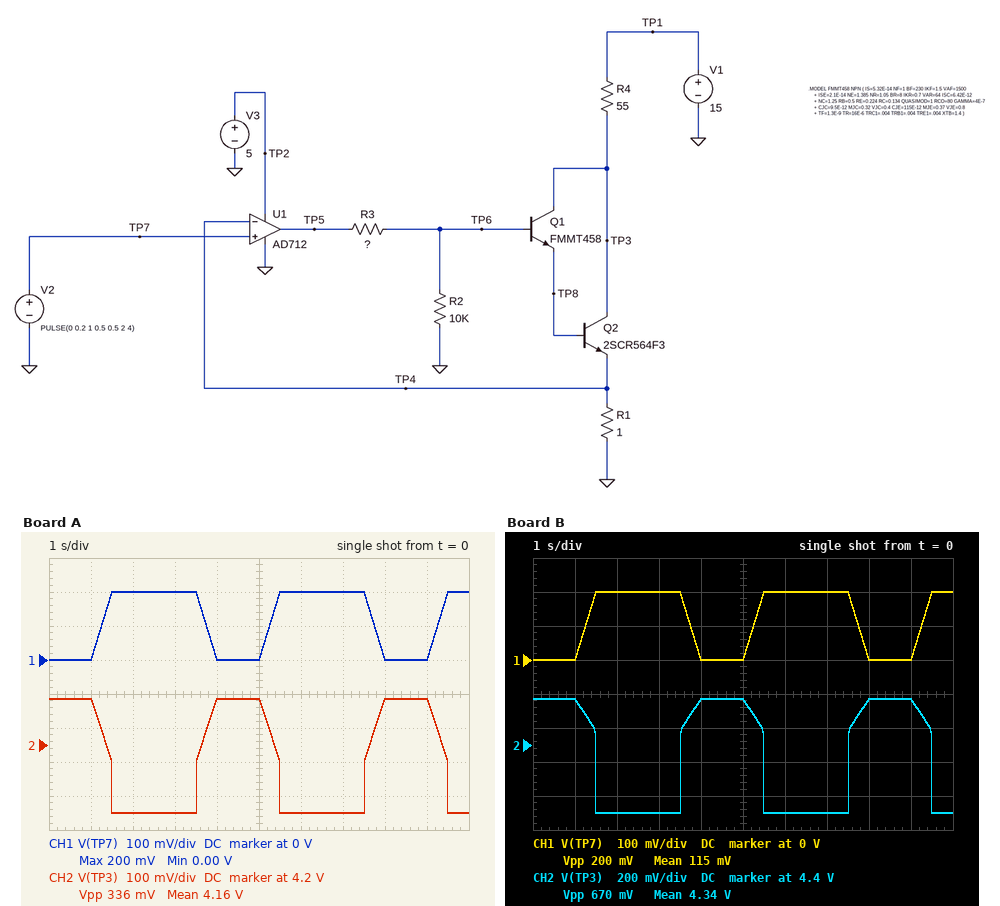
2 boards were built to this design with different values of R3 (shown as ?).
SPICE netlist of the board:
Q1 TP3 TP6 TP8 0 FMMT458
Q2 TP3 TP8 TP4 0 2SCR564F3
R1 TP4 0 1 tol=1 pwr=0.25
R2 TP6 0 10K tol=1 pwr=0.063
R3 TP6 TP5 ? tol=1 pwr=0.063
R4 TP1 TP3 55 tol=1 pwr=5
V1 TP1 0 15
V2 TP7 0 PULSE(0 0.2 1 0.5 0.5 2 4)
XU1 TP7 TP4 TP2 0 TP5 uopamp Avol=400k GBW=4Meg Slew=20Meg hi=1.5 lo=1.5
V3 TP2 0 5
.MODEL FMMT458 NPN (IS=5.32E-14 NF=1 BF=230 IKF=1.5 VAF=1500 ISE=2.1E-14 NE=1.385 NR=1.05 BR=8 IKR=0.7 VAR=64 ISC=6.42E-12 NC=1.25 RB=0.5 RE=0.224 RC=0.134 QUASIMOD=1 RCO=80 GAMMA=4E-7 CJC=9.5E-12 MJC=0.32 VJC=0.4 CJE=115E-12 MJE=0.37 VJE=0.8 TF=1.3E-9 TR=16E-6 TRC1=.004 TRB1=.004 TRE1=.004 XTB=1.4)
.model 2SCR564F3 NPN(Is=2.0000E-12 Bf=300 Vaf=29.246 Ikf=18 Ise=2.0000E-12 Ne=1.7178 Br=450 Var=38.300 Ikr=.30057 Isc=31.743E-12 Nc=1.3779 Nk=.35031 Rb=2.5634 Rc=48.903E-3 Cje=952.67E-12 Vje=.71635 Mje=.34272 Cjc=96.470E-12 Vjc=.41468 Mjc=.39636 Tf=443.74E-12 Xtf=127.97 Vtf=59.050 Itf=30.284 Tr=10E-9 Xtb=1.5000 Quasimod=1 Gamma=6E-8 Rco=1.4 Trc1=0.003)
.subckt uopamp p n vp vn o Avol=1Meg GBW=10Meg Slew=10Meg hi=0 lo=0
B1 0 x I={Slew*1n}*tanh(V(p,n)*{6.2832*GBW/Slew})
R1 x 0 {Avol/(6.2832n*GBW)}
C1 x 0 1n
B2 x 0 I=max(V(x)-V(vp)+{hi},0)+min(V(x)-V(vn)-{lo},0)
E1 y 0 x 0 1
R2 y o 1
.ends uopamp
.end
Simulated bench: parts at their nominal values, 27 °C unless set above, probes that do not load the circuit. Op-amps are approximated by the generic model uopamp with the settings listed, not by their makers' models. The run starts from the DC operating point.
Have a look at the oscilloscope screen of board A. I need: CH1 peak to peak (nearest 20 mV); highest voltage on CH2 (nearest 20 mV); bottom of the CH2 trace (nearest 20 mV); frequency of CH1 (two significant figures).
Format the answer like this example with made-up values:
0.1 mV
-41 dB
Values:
200 mV
4.34 V
4.00 V
250 mHz
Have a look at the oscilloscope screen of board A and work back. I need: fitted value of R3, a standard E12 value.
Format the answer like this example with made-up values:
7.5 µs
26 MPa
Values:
330 Ω
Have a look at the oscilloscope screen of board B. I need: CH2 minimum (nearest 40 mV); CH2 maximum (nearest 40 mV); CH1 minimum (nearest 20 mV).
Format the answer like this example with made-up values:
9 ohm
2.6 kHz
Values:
4.00 V
4.68 V
0 V
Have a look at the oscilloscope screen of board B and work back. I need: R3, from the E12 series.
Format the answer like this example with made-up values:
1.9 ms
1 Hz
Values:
390 Ω
